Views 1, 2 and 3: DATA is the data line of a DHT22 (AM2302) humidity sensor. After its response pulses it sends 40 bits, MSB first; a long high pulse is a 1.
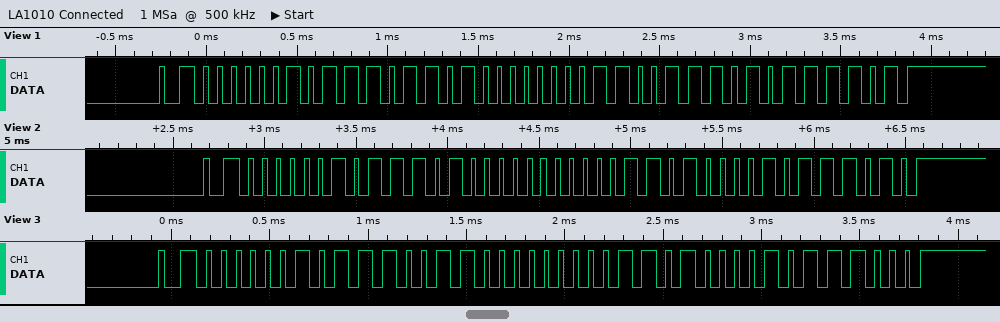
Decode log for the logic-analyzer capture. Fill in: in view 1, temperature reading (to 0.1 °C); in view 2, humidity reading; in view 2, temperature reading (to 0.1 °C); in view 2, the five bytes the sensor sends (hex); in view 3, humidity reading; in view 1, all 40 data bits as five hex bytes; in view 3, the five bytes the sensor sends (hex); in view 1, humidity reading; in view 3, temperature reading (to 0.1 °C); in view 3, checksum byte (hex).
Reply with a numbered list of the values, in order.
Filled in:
1. 20.6 °C
2. 74.4 %
3. 20.8 °C
4. 02 E8 00 D0 BA
5. 74.2 %
6. 02 ED 00 CE BD
7. 02 E6 00 D0 B8
8. 74.9 %
9. 20.8 °C
10. 0xB8
